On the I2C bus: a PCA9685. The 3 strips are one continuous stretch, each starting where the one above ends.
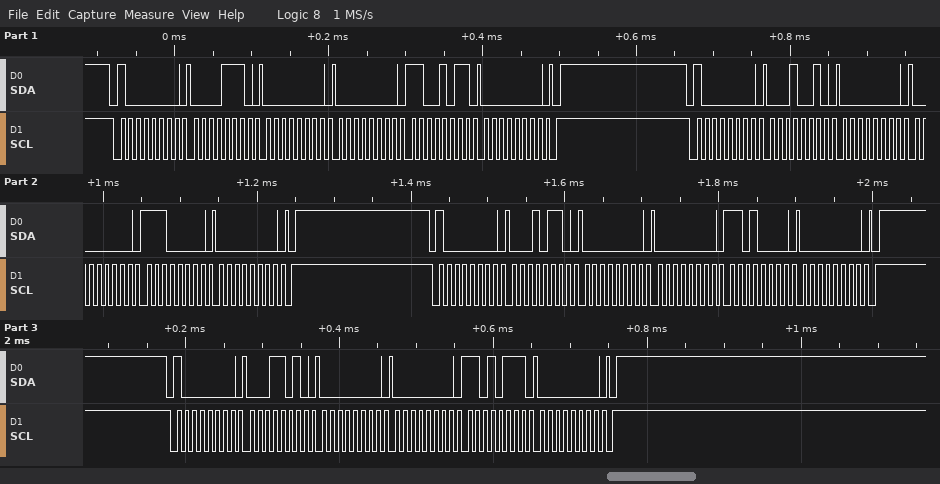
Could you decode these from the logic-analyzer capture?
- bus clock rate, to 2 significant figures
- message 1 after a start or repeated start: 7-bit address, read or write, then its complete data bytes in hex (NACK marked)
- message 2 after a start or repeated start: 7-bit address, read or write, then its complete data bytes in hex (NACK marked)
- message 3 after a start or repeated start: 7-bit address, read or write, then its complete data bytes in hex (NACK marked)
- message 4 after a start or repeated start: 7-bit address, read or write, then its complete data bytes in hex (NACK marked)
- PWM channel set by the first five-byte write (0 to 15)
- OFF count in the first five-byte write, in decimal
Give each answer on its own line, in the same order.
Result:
100 kHz
0x40 write: 0E 00 00 CB 00
0x40 write: 12 00 00 E0 00
0x40 write: 16 00 00 D0 00
0x40 write: 1A 00 00 D7 00
2
203
